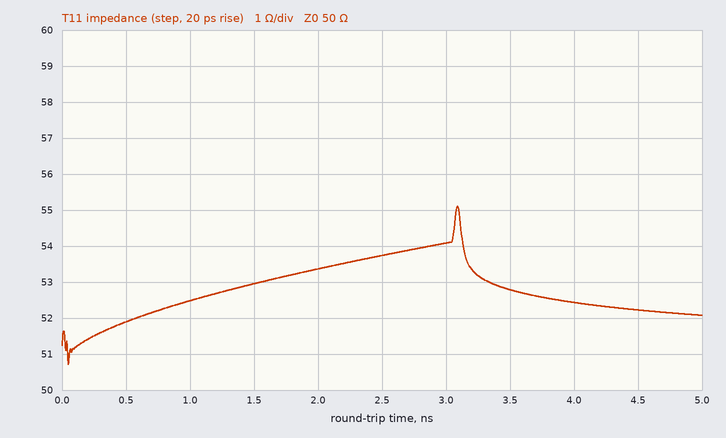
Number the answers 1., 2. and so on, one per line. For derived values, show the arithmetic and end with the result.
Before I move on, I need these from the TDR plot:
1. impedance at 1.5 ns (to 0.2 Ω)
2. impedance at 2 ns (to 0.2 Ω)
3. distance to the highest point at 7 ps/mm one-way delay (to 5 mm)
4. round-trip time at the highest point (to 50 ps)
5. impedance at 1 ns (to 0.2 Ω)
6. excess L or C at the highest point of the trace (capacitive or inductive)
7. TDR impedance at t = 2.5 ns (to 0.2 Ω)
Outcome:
1. 53.0 Ω
2. 53.4 Ω
3. 3.10 ns / 2 / 7 ps/mm ≈ 221 mm, so 220 mm to the nearest 5 mm
4. 3.10 ns
5. 52.4 Ω
6. inductive
7. 53.8 Ω
